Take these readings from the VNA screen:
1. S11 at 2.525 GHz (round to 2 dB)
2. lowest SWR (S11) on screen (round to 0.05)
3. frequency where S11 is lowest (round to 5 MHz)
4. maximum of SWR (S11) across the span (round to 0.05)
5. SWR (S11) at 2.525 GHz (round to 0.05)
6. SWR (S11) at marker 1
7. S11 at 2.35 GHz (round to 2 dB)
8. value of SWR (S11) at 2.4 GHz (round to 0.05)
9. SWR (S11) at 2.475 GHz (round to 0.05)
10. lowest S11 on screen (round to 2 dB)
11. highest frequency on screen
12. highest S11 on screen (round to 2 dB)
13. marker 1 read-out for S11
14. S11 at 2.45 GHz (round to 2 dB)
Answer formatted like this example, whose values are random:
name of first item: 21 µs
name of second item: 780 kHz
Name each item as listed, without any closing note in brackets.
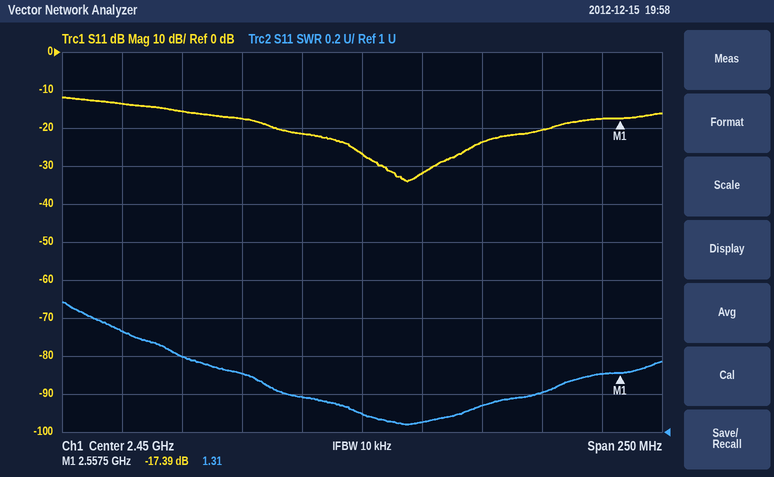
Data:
S11 at 2.525 GHz: -20 dB
lowest SWR (S11) on screen: 1.05
frequency where S11 is lowest: 2.470 GHz
maximum of SWR (S11) across the span: 1.70
SWR (S11) at 2.525 GHz: 1.20
SWR (S11) at marker 1: 1.31
S11 at 2.35 GHz: -14 dB
value of SWR (S11) at 2.4 GHz: 1.30
SWR (S11) at 2.475 GHz: 1.05
lowest S11 on screen: -34 dB
highest frequency on screen: 2.575 GHz
highest S11 on screen: -12 dB
marker 1 read-out for S11: -17.39 dB
S11 at 2.45 GHz: -26 dB
